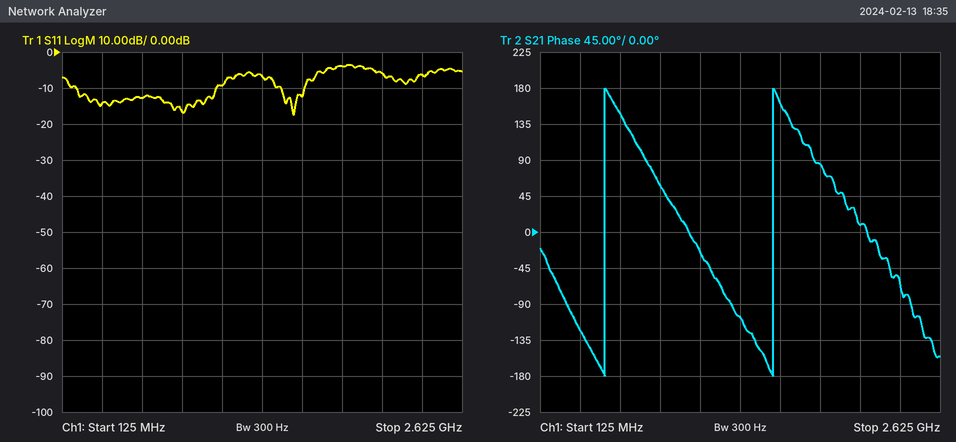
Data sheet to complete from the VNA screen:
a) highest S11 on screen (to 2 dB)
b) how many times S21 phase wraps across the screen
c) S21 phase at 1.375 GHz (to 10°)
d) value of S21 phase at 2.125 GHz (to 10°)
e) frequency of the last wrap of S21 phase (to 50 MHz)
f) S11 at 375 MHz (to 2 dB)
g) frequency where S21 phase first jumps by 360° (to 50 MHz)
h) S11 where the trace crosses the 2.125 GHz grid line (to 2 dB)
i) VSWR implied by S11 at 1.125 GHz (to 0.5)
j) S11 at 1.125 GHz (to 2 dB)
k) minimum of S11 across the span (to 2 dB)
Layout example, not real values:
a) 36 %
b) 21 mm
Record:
a) -4 dB
b) 2
c) -110°
d) 10°
e) 1.60 GHz
f) -14 dB
g) 550 MHz
h) -6 dB
i) 2.0
j) -10 dB
k) -18 dB
